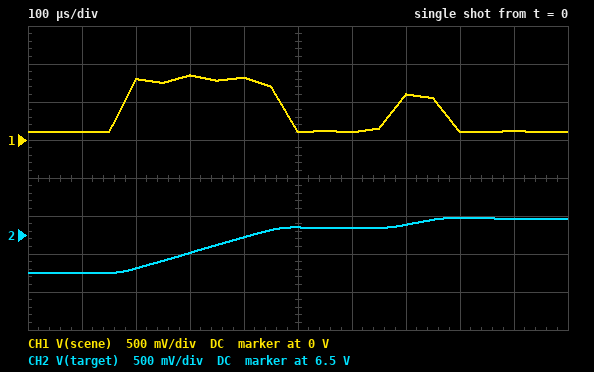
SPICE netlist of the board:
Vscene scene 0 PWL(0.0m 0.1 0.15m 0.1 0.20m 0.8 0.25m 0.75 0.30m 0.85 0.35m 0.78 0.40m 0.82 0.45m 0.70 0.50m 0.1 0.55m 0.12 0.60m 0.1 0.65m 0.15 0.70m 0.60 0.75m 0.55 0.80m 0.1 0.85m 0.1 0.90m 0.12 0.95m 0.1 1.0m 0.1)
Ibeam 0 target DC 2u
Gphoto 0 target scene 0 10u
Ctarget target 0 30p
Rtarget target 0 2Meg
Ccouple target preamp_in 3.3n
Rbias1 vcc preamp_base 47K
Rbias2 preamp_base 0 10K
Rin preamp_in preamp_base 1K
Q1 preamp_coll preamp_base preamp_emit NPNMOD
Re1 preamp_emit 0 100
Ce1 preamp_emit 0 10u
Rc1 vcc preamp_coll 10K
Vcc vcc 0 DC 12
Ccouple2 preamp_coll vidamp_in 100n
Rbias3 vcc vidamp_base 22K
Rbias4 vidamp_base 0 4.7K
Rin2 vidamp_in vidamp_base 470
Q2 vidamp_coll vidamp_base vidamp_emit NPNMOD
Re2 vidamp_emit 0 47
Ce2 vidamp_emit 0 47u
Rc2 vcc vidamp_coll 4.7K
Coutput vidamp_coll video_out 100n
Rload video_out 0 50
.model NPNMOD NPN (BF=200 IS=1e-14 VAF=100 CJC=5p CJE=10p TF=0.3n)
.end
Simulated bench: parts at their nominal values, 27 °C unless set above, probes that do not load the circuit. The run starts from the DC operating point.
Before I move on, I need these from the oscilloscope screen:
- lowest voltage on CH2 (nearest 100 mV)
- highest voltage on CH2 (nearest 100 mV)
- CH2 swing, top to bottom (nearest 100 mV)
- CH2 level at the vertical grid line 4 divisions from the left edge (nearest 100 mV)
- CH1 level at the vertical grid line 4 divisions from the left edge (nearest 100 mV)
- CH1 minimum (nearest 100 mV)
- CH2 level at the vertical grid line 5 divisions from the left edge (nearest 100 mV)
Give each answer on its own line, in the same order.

6.0 V
6.7 V
700 mV
6.5 V
800 mV
100 mV
6.6 V
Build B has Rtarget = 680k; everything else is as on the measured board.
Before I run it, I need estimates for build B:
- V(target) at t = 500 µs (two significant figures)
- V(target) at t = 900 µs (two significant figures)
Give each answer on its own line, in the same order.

2.6 V
2.7 V
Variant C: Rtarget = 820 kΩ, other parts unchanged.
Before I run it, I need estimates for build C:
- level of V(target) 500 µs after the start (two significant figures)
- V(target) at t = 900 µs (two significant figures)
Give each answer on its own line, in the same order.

3.0 V
3.1 V
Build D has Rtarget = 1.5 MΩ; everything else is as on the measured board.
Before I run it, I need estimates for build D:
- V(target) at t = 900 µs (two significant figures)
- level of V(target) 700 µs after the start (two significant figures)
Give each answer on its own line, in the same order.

5.2 V
5.1 V
